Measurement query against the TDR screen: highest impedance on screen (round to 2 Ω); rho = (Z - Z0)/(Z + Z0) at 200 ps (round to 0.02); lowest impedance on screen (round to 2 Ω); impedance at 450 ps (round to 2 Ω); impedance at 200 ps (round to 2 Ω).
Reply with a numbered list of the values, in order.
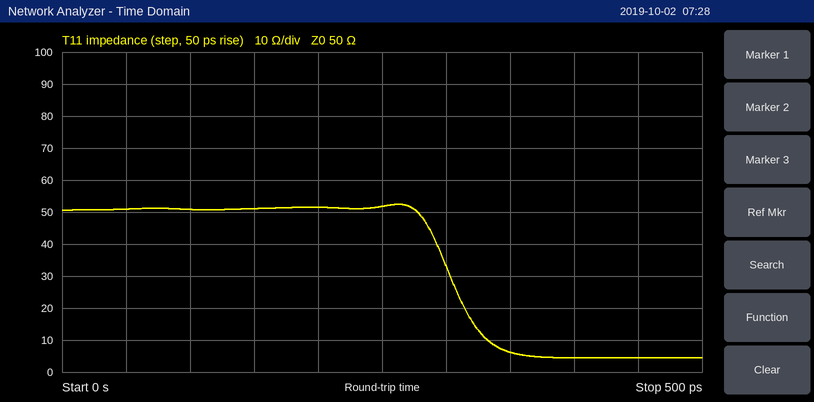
1. 52 Ω
2. +0.02
3. 4 Ω
4. 4 Ω
5. 52 Ω
